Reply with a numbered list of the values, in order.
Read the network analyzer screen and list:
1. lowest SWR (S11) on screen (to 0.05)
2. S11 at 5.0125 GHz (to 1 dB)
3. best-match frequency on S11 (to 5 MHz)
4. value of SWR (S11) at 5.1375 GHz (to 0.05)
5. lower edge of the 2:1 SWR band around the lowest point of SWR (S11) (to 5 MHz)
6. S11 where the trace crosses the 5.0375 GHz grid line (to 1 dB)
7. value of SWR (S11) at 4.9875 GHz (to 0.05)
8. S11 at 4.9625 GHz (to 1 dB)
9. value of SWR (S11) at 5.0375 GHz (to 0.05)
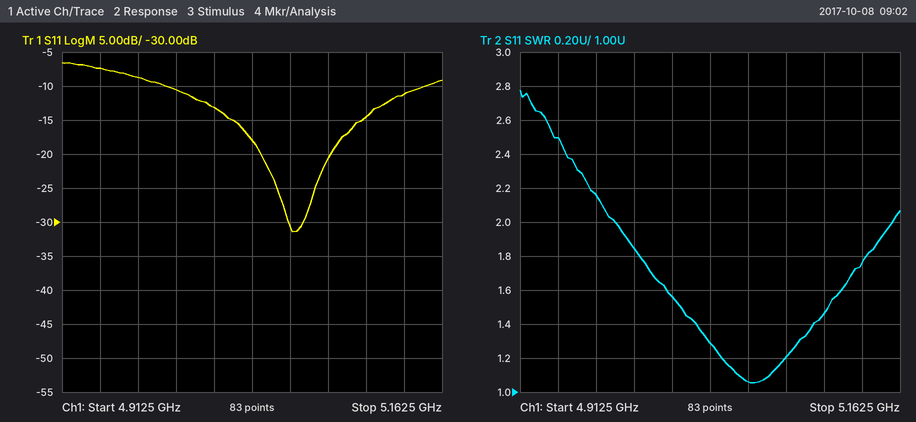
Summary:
1. 1.05
2. -13 dB
3. 5.065 GHz
4. 1.75
5. 4.975 GHz
6. -18 dB
7. 1.85
8. -9 dB
9. 1.30
